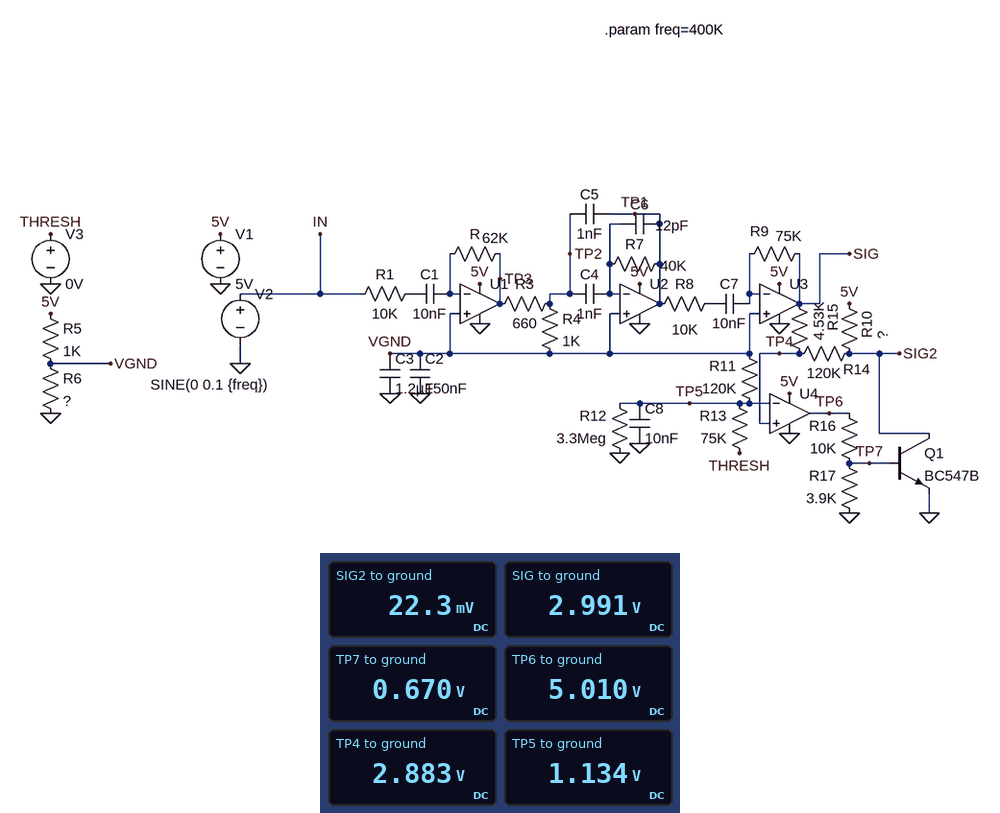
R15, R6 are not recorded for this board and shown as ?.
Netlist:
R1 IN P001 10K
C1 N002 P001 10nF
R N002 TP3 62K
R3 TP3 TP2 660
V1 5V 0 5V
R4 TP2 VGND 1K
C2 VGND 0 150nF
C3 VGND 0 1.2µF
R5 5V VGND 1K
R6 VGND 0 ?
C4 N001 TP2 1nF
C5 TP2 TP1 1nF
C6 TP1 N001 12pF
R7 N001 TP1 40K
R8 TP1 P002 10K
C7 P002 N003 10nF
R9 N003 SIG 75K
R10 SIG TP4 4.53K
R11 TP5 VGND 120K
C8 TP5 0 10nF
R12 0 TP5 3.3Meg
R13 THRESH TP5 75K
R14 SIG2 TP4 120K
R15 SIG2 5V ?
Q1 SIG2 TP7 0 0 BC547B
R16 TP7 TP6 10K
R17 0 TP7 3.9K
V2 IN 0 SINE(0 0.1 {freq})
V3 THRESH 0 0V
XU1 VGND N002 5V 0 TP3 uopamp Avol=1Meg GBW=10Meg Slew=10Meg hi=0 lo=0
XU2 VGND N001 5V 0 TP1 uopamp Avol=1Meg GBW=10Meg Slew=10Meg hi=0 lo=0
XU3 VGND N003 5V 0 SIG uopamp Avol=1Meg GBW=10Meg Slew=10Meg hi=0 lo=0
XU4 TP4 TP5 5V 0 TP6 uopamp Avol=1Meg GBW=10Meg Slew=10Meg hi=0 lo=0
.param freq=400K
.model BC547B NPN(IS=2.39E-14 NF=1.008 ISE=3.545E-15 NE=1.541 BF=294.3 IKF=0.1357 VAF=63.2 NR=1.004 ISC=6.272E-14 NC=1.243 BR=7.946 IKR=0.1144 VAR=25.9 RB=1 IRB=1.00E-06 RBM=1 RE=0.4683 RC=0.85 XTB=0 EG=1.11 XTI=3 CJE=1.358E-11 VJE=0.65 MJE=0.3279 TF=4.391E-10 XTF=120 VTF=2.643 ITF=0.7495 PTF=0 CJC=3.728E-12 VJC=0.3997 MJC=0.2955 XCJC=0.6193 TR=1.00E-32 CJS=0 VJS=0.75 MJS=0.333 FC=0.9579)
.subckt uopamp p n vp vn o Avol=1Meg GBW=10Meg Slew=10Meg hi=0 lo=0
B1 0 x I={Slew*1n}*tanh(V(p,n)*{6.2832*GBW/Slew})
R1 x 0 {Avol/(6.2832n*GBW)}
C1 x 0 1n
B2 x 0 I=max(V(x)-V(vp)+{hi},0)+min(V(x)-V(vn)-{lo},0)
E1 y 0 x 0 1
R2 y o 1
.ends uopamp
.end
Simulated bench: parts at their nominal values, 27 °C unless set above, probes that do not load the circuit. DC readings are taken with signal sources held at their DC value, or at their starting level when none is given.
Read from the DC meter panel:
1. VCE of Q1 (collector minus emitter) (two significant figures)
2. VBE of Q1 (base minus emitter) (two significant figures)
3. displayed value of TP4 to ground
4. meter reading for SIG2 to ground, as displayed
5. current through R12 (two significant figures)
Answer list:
22 mV
670 mV
2.883 V
22.3 mV
340 nA
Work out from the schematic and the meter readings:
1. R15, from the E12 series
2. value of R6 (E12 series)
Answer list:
3.9 kΩ
1.5 kΩ
